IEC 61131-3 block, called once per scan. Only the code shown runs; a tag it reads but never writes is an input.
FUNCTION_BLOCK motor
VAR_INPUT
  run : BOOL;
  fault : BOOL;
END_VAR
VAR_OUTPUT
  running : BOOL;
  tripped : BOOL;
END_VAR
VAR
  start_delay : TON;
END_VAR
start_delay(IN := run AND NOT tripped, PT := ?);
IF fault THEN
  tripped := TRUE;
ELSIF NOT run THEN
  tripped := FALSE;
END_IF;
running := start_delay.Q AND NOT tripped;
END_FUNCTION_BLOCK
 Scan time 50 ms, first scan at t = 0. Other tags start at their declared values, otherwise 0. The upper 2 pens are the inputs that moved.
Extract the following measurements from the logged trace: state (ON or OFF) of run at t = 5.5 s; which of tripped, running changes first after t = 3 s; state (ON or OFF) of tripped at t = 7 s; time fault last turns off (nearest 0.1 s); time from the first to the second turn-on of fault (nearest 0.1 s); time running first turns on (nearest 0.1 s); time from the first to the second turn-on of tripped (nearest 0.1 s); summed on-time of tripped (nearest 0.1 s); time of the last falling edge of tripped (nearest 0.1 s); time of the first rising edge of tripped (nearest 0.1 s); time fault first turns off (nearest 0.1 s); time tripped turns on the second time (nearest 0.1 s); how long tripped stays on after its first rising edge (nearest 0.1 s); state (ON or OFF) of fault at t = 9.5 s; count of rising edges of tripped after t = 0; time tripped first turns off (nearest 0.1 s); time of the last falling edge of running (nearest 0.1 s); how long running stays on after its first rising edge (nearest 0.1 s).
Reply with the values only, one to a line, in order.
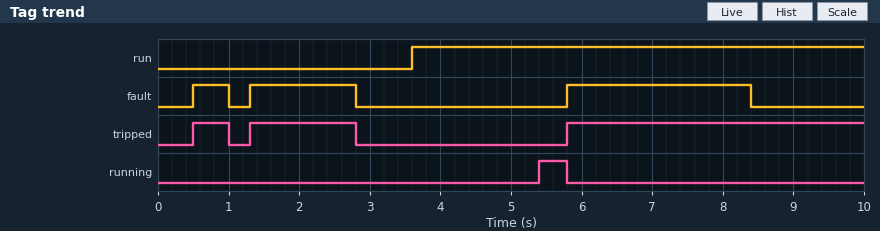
ON
running
ON
8.4 s
0.8 s
5.4 s
0.8 s
6.2 s
2.8 s
0.5 s
1.0 s
1.3 s
0.5 s
OFF
3
1.0 s
5.8 s
0.4 s
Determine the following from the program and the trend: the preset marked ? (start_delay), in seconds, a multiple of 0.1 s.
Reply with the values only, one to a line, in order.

1.8 s
